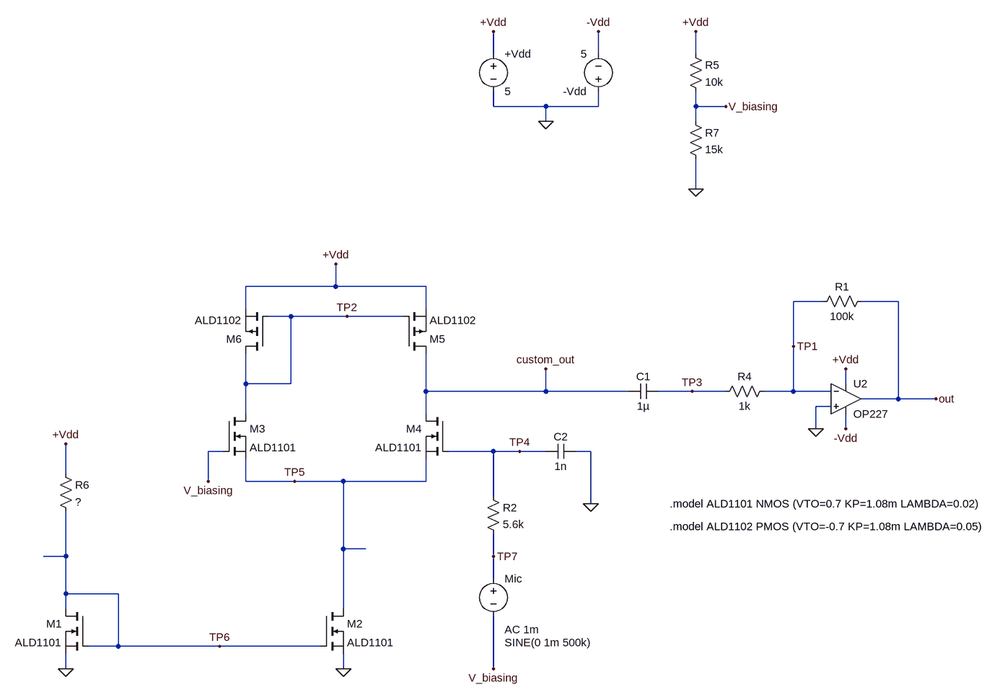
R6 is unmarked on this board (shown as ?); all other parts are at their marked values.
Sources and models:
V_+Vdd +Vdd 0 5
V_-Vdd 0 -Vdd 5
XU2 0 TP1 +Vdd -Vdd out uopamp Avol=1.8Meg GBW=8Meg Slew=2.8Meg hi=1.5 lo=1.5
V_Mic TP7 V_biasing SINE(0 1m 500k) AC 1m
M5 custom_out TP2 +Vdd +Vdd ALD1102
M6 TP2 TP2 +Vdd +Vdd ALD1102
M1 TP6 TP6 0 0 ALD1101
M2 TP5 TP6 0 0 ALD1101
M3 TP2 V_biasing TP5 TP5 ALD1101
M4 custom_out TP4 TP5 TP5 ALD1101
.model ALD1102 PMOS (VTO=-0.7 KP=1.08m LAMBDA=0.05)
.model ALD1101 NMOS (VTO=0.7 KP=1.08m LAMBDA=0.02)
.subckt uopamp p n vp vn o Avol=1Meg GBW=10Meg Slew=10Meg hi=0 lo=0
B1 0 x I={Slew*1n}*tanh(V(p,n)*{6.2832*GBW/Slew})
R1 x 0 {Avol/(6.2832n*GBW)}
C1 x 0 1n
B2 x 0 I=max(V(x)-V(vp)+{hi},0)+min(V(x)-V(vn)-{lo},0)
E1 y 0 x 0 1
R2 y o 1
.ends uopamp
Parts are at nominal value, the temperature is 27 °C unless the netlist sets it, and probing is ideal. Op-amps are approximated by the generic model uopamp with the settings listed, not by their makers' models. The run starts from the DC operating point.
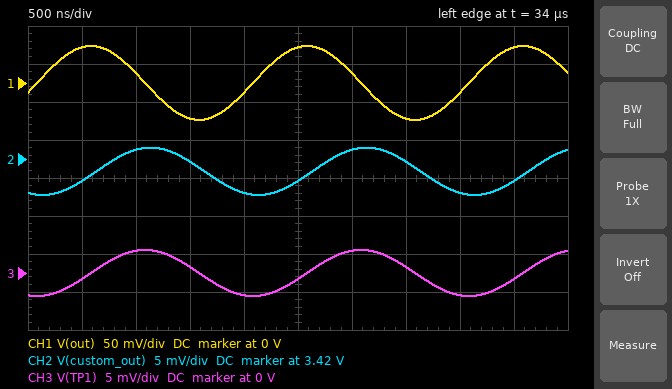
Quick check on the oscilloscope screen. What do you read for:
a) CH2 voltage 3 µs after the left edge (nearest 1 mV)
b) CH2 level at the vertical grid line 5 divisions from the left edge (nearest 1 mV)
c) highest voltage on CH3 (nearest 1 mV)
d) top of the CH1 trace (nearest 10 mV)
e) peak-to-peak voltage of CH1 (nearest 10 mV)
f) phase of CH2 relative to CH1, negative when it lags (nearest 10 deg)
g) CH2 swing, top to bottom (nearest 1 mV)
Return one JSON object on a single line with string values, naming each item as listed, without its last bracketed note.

{"CH2 voltage 3 µs after the left edge": "3.421 V", "CH2 level at the vertical grid line 5 divisions from the left edge": "3.417 V", "highest voltage on CH3": "3 mV", "top of the CH1 trace": "50 mV", "peak-to-peak voltage of CH1": "100 mV", "phase of CH2 relative to CH1, negative when it lags": "-100 deg", "CH2 swing, top to bottom": "6 mV"}
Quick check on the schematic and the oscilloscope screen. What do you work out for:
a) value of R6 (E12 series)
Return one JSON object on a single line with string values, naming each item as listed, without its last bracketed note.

{"value of R6": "3.3 kΩ"}
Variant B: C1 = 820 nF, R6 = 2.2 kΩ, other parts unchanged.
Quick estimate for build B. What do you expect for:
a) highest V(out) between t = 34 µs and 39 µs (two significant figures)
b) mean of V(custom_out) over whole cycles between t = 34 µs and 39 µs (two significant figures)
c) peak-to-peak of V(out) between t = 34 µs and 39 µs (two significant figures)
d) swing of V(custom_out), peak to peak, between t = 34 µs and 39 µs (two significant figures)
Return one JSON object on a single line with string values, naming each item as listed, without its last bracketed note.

{"highest V(out) between t = 34 µs and 39 µs": "55 mV", "mean of V(custom_out) over whole cycles between t = 34 µs and 39 µs": "3.3 V", "peak-to-peak of V(out) between t = 34 µs and 39 µs": "110 mV", "swing of V(custom_out), peak to peak, between t = 34 µs and 39 µs": "7.0 mV"}
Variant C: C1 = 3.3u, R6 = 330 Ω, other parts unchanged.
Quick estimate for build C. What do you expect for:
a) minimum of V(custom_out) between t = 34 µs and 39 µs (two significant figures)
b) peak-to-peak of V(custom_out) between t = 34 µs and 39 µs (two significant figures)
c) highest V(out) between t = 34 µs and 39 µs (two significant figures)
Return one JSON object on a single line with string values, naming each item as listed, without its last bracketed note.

{"minimum of V(custom_out) between t = 34 µs and 39 µs": "2.9 V", "peak-to-peak of V(custom_out) between t = 34 µs and 39 µs": "8.6 mV", "highest V(out) between t = 34 µs and 39 µs": "67 mV"}
